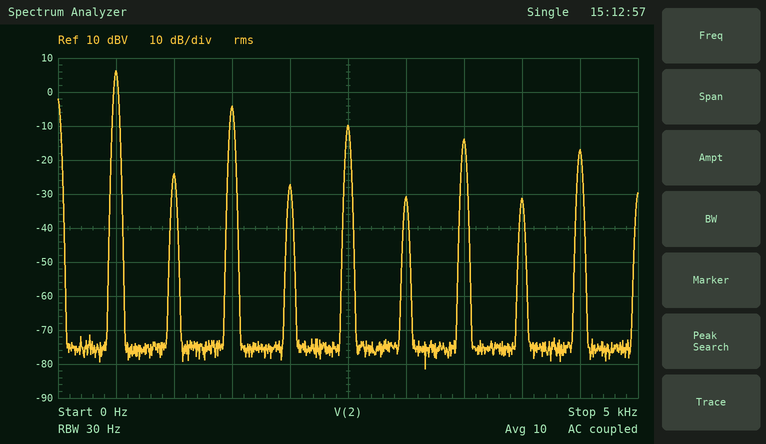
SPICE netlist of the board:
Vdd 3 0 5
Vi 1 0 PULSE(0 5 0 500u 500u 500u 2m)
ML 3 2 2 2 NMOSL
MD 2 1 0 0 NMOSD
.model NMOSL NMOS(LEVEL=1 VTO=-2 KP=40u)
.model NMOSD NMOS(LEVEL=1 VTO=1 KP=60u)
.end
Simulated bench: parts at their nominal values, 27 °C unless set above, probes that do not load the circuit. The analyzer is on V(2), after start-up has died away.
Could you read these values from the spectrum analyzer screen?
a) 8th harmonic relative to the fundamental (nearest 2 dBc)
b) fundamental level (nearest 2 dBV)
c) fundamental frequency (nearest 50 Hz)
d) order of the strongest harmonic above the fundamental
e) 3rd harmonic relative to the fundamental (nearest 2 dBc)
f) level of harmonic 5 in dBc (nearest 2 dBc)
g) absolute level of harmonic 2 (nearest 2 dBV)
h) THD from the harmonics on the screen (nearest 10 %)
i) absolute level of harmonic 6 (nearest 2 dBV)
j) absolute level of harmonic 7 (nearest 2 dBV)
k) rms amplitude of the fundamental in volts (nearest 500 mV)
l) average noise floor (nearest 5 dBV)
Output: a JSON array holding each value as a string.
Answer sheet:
["-38 dBc", "6 dBV", "500 Hz", "3", "-10 dBc", "-16 dBc", "-24 dBV", "40 %", "-30 dBV", "-14 dBV", "2.0 V", "-75 dBV"]
